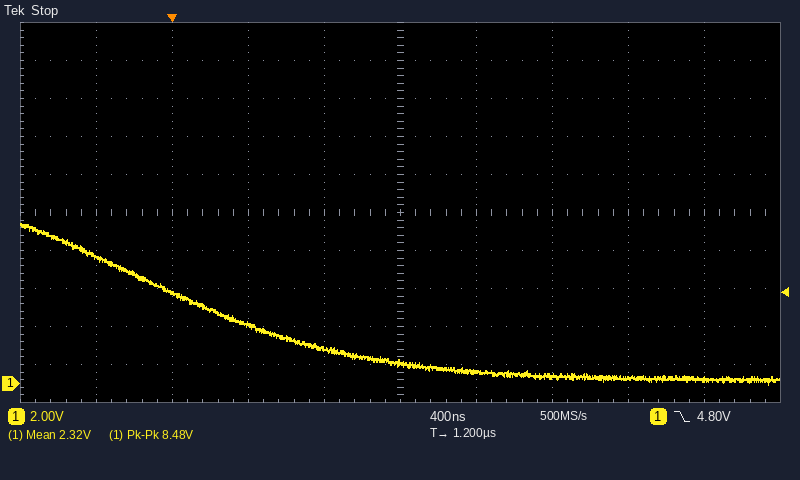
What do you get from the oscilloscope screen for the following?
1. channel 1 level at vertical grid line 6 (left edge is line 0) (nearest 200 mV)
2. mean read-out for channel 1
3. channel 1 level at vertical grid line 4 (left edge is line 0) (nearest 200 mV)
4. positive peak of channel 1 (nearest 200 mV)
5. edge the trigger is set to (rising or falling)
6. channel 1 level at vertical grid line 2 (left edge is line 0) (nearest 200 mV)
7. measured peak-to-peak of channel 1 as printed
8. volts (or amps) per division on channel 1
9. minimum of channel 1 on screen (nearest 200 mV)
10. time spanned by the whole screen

600 mV
2.32 V
1.8 V
8.4 V
falling
4.8 V
8.48 V
2 V
0.0 V
4 µs
